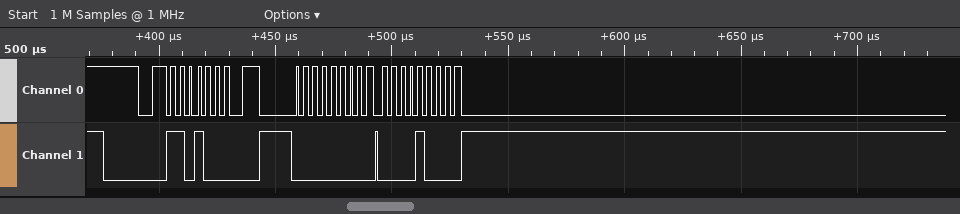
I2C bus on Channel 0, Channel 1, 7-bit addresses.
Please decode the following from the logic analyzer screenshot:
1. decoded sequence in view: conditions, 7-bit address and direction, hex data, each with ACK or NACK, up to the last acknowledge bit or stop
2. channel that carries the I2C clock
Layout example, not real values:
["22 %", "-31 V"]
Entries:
["start, address 34 write ACK, 00 ACK, 08 ACK", "Channel 0"]
